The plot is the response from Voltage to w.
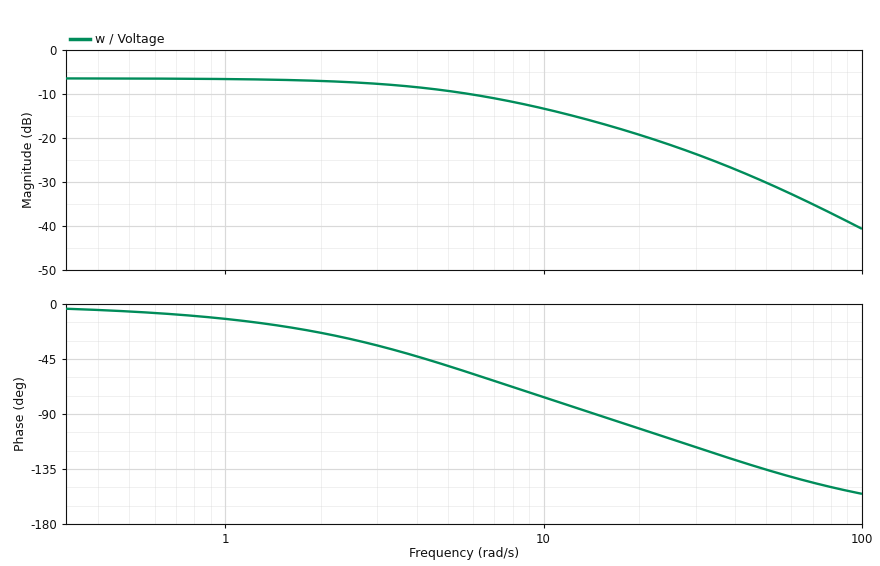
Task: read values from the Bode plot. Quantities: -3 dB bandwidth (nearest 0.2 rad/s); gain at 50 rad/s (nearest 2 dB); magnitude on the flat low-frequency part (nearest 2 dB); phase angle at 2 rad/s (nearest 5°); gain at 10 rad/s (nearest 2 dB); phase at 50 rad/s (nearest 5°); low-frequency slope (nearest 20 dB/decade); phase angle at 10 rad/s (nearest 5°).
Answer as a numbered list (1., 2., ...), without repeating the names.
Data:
1. 5.2 rad/s
2. -30 dB
3. -6 dB
4. -25°
5. -14 dB
6. -135°
7. 0 dB/decade
8. -75°
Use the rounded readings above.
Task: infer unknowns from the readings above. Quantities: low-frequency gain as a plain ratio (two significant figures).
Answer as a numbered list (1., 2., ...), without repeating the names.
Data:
1. 0.50
